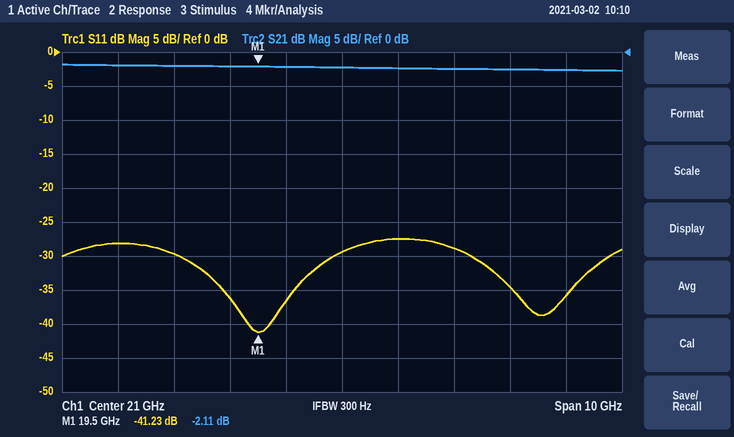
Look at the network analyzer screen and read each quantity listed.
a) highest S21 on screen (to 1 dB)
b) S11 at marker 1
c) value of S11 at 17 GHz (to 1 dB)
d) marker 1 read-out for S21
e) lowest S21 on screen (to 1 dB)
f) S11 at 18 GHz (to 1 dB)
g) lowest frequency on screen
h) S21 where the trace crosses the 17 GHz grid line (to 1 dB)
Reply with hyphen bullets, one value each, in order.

- -2 dB
- -41.23 dB
- -28 dB
- -2.11 dB
- -3 dB
- -30 dB
- 16 GHz
- -2 dB
